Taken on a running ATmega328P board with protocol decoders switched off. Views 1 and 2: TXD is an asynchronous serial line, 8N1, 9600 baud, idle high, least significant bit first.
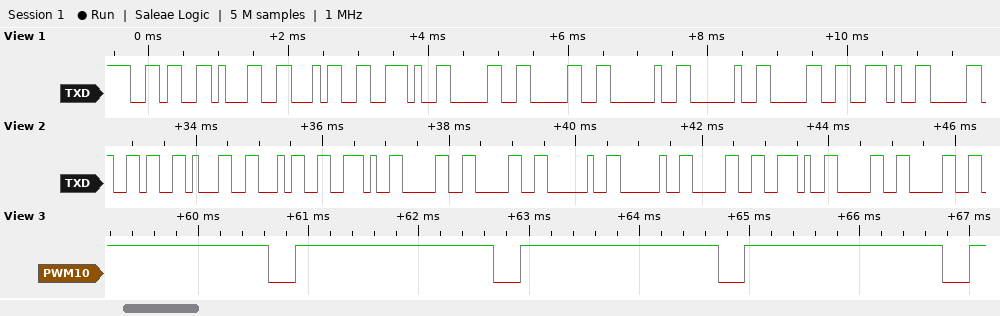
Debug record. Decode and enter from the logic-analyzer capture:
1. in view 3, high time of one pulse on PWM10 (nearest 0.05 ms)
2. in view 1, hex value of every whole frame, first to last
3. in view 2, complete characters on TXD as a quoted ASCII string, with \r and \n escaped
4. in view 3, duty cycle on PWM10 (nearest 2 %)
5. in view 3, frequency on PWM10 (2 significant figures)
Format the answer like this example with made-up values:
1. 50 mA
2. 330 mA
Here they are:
1. 1.80 ms
2. 0x36 0x31 0x34 0x2E 0x30 0x30 0x20 0x20 0x30 0x2E
3. "614.00  0.00"
4. 88 %
5. 490 Hz
